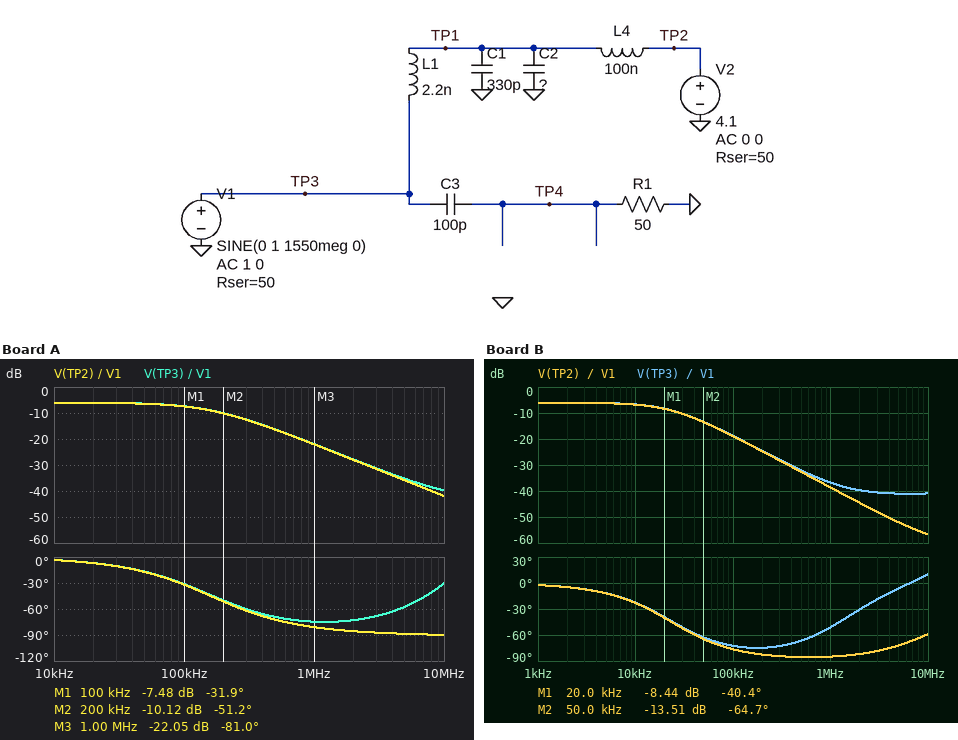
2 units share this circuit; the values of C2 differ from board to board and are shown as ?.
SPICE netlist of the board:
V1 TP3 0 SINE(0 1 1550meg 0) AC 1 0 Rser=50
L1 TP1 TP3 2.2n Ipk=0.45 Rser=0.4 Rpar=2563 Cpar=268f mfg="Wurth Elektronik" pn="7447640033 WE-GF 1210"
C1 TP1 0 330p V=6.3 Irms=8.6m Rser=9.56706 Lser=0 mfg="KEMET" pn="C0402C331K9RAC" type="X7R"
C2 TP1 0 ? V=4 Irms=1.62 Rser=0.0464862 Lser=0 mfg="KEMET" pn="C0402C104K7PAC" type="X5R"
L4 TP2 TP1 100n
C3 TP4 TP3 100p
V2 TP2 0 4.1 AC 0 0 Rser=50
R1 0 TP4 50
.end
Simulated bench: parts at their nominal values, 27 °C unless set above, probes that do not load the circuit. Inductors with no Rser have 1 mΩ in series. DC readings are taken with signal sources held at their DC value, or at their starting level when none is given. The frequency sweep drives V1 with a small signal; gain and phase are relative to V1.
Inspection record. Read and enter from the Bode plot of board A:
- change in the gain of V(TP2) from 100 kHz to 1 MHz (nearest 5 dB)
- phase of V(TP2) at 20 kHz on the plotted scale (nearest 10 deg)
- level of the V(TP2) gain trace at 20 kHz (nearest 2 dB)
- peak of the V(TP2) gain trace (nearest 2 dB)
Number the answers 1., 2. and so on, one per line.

1. -15 dB
2. -10 deg
3. -6 dB
4. -6 dB
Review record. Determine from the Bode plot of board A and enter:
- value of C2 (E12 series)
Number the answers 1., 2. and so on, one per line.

1. 39 nF
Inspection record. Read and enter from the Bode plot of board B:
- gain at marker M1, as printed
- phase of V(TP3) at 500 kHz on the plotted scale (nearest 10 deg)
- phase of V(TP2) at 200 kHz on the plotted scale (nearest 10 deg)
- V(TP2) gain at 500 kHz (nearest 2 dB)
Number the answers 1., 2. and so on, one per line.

1. -8.44 dB
2. -70 deg
3. -80 deg
4. -32 dB
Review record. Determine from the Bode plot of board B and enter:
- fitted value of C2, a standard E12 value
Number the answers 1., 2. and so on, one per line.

1. 270 nF
